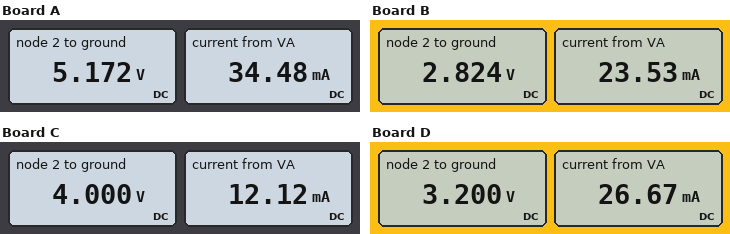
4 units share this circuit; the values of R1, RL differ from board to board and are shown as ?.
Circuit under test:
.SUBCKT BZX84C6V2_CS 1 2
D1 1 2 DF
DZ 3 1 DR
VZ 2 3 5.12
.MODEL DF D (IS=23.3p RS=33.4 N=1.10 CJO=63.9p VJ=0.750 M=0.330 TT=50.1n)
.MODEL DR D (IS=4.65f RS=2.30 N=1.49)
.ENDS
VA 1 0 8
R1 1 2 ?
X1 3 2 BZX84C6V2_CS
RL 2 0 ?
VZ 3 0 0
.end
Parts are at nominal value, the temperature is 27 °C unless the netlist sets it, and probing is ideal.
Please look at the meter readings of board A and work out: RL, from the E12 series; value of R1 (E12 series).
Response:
150 Ω
82 Ω
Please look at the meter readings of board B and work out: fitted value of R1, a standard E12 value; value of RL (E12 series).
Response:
220 Ω
120 Ω
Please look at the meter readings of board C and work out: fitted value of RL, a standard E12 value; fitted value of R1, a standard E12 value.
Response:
330 Ω
330 Ω
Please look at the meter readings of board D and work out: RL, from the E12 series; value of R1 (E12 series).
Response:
120 Ω
180 Ω
